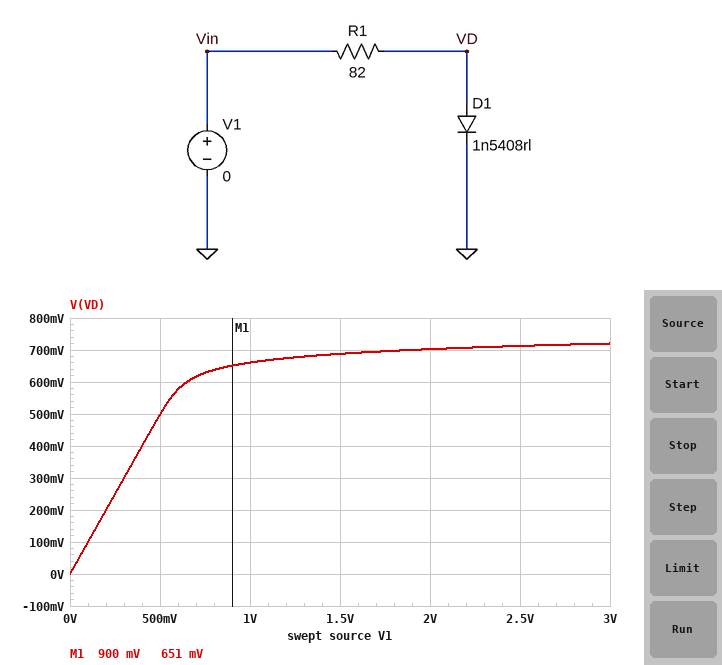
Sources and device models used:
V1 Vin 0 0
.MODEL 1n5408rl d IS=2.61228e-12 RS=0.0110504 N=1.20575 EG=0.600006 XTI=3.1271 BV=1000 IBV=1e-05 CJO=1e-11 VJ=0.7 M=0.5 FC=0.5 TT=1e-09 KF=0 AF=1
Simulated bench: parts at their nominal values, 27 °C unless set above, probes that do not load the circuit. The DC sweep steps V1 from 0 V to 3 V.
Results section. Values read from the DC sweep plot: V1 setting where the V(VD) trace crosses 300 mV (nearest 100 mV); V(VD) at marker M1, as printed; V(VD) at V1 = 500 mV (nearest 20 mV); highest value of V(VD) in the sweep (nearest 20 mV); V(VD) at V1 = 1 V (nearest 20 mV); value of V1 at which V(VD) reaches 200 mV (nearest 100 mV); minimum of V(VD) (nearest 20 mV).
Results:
300 mV
651 mV
500 mV
720 mV
660 mV
200 mV
0 V
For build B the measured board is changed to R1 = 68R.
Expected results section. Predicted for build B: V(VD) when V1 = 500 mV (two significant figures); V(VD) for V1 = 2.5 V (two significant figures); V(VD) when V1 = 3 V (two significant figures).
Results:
500 mV
720 mV
730 mV
